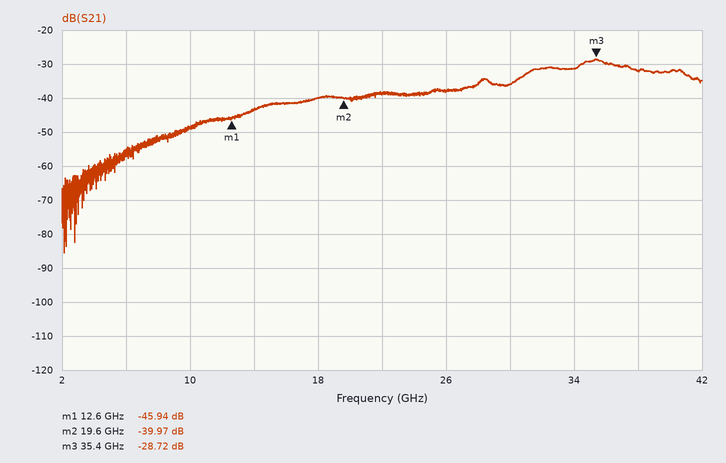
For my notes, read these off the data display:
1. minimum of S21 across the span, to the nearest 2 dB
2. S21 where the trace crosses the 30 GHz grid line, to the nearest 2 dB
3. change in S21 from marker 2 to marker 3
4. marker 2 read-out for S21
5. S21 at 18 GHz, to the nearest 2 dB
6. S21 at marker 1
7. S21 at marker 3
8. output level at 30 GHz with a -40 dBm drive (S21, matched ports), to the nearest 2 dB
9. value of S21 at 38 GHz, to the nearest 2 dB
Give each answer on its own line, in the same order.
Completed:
-86 dB
-36 dB
11.25 dB
-39.97 dB
-40 dB
-45.94 dB
-28.72 dB
-76 dBm
-32 dB
